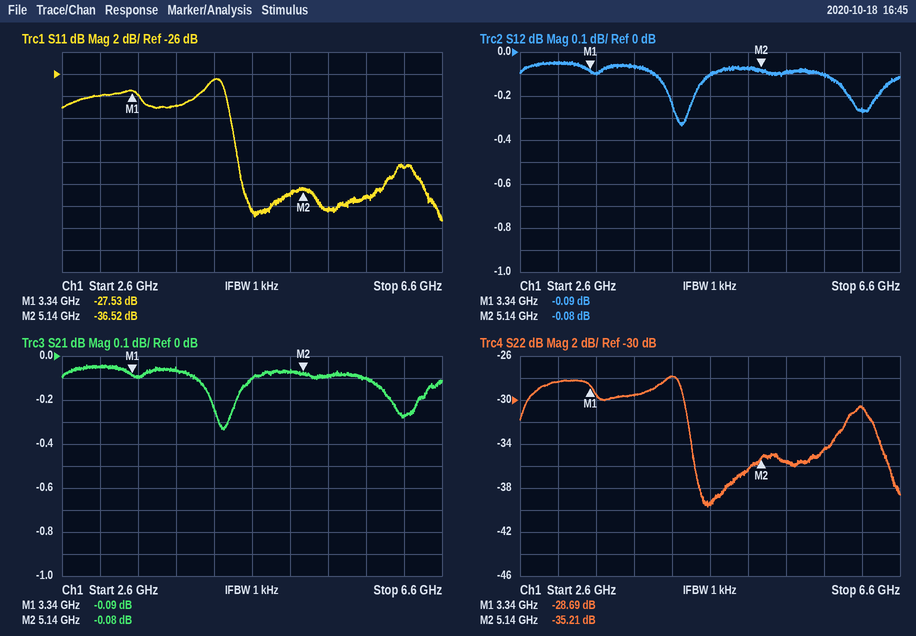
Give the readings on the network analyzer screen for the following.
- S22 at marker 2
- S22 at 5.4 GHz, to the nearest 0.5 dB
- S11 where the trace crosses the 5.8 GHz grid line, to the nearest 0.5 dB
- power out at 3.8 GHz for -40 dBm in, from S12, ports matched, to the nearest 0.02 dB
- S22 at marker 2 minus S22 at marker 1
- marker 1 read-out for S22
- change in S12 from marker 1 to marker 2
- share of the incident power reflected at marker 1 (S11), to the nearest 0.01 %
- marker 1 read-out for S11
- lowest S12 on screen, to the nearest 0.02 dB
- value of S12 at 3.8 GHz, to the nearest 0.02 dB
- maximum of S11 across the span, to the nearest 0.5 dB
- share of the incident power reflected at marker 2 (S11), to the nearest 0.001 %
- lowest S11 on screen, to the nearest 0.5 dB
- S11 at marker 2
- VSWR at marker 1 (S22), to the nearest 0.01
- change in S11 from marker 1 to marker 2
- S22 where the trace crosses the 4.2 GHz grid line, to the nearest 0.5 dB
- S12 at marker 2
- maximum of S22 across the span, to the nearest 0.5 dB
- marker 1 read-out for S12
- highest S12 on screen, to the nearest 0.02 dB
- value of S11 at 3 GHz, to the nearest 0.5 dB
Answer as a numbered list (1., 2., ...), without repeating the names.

1. -35.21 dB
2. -35.5 dB
3. -37.0 dB
4. -40.06 dBm
5. -6.52 dB
6. -28.69 dB
7. 0.01 dB
8. 0.18 %
9. -27.53 dB
10. -0.34 dB
11. -0.06 dB
12. -26.5 dB
13. 0.022 %
14. -39.5 dB
15. -36.52 dB
16. 1.08
17. -8.99 dB
18. -28.0 dB
19. -0.08 dB
20. -28.0 dB
21. -0.09 dB
22. -0.04 dB
23. -28.0 dB
